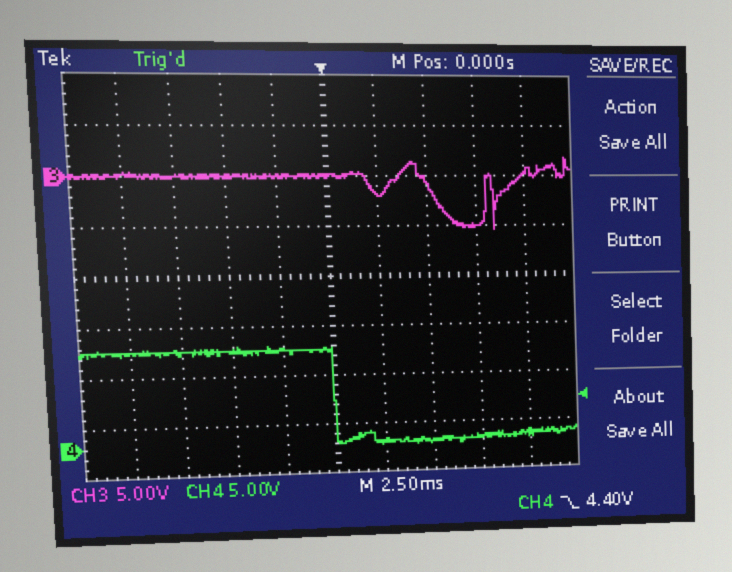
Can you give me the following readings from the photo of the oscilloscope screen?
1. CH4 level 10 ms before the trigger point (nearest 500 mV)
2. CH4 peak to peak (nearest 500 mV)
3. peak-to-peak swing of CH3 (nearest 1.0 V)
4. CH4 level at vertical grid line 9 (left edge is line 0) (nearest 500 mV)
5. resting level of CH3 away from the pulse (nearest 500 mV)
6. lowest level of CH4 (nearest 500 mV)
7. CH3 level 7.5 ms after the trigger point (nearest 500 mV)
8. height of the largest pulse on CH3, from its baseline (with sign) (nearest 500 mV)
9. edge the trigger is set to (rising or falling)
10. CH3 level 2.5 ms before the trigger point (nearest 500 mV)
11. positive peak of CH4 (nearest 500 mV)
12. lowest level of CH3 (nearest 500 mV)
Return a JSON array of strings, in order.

["9.5 V", "10.0 V", "7.0 V", "500 mV", "0.0 V", "0.0 V", "-5.0 V", "-5.5 V", "falling", "0.0 V", "10.0 V", "-5.5 V"]
